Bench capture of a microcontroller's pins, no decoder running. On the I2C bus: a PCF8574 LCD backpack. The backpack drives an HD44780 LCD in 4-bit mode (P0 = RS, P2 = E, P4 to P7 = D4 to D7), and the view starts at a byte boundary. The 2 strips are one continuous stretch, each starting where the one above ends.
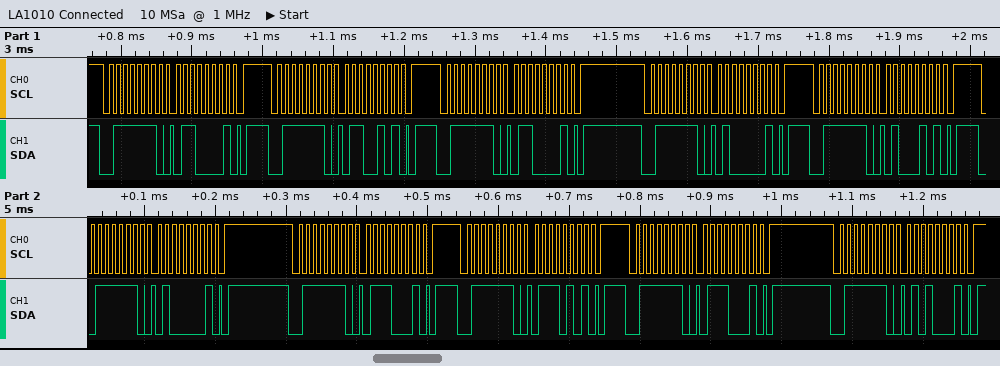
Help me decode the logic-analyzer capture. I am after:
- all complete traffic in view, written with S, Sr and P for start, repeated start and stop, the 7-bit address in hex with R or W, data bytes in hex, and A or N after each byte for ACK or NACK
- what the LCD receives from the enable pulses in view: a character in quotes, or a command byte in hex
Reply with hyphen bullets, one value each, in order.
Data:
- S 3FW A 61 A P S 3FW A 65 A P S 3FW A 61 A P S 3FW A 41 A P S 3FW A 45 A P S 3FW A 41 A P S 3FW A 71 A P S 3FW A 75 A P S 3FW A 71 A P S 3FW A 51 A P
- 'd'
